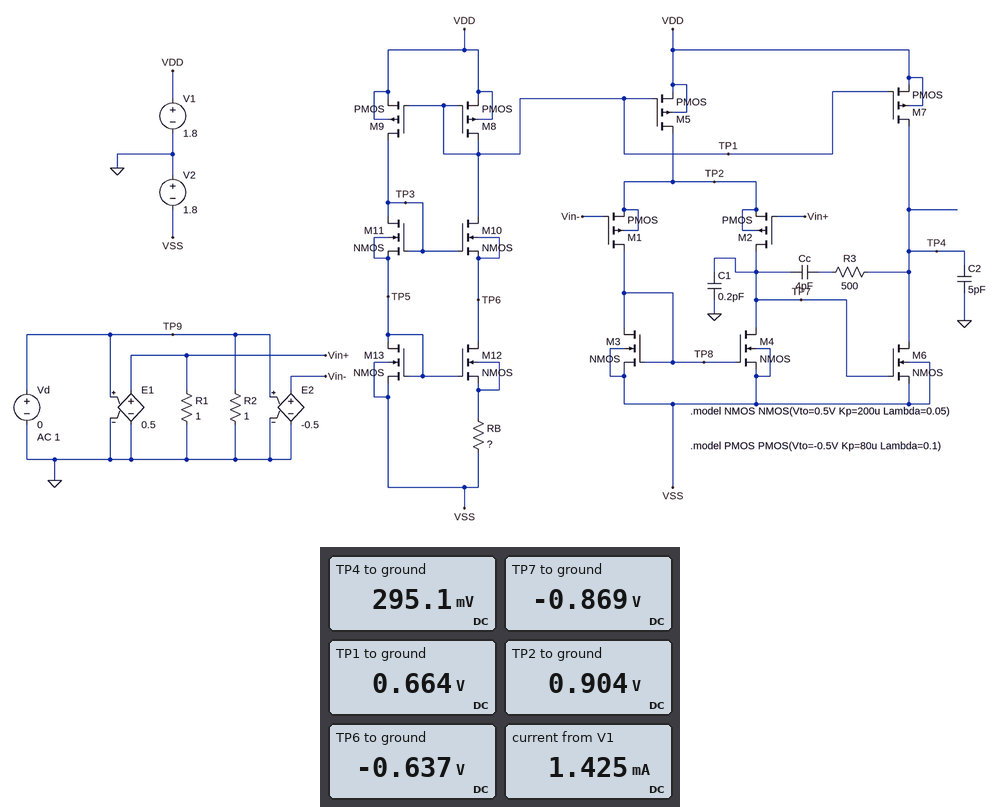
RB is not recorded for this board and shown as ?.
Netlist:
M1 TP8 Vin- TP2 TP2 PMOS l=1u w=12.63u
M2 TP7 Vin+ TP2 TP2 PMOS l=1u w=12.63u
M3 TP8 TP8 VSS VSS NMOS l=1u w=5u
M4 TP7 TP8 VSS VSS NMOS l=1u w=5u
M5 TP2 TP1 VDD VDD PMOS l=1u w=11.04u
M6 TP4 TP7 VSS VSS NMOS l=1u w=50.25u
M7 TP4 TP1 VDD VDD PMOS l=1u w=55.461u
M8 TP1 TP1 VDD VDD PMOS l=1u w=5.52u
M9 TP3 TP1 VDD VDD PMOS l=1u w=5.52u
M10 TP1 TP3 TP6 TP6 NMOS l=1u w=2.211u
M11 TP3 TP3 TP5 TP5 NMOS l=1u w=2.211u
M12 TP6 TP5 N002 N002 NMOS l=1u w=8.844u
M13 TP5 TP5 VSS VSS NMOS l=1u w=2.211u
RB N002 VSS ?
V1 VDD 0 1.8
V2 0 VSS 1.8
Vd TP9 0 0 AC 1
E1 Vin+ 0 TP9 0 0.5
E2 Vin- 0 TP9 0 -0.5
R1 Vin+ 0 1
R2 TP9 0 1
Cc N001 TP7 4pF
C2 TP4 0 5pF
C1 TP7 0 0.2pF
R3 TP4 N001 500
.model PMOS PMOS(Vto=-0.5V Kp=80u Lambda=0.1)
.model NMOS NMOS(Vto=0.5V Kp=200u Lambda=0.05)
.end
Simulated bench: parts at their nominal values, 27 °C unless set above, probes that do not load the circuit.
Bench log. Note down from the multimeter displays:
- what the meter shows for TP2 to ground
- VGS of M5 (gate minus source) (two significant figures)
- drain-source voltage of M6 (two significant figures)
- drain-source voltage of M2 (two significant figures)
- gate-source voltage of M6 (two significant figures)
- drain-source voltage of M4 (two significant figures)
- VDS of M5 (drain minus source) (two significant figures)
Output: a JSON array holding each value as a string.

["0.904 V", "-1.1 V", "2.1 V", "-1.8 V", "930 mV", "930 mV", "-900 mV"]
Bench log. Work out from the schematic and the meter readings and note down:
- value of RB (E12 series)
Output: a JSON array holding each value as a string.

["3.3 kΩ"]
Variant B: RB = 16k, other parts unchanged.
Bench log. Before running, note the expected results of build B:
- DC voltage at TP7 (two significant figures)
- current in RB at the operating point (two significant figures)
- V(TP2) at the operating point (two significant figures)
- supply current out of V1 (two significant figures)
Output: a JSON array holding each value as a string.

["-1.2 V", "5.6 µA", "600 mV", "86 µA"]
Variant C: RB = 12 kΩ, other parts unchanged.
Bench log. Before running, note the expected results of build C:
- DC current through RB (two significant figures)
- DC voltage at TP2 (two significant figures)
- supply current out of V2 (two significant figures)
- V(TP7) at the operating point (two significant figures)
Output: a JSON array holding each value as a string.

["9.7 µA", "630 mV", "150 µA", "-1.2 V"]
